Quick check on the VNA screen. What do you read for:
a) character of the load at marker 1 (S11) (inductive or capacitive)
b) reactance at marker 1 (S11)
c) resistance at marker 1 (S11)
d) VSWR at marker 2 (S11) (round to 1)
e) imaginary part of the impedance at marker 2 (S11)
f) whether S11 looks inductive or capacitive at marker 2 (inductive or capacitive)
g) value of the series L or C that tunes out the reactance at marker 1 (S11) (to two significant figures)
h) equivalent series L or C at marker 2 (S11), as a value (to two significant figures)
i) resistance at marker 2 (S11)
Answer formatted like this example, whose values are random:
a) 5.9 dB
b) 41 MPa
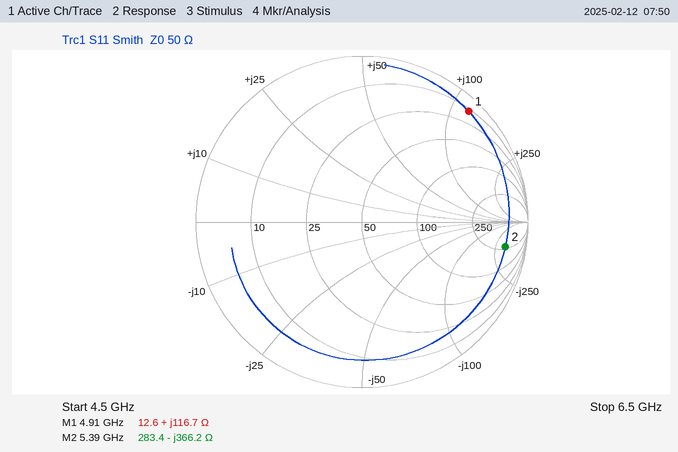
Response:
a) inductive
b) +116.7 Ω
c) 12.6 Ω
d) 15
e) -366.2 Ω
f) capacitive
g) 280 fF
h) 81 fF
i) 283.4 Ω
